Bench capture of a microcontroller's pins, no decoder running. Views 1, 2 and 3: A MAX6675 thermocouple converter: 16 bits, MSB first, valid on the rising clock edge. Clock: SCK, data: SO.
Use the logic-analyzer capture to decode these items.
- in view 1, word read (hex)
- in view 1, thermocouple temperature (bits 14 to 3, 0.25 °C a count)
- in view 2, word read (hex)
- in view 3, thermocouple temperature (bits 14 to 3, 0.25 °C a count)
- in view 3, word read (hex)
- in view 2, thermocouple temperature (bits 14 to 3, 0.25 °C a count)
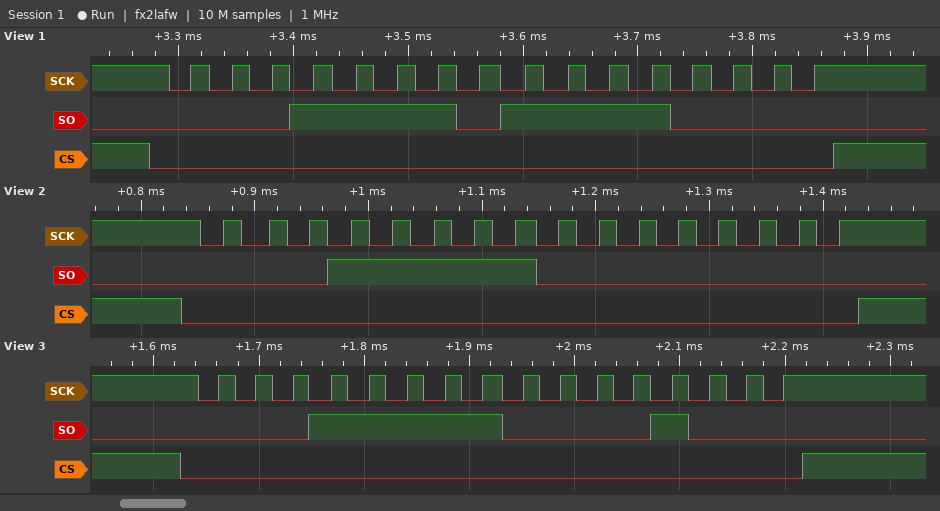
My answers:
0x1EF0
247.50 °C
0x1F00
248.25 °C
0x1F08
248.00 °C
